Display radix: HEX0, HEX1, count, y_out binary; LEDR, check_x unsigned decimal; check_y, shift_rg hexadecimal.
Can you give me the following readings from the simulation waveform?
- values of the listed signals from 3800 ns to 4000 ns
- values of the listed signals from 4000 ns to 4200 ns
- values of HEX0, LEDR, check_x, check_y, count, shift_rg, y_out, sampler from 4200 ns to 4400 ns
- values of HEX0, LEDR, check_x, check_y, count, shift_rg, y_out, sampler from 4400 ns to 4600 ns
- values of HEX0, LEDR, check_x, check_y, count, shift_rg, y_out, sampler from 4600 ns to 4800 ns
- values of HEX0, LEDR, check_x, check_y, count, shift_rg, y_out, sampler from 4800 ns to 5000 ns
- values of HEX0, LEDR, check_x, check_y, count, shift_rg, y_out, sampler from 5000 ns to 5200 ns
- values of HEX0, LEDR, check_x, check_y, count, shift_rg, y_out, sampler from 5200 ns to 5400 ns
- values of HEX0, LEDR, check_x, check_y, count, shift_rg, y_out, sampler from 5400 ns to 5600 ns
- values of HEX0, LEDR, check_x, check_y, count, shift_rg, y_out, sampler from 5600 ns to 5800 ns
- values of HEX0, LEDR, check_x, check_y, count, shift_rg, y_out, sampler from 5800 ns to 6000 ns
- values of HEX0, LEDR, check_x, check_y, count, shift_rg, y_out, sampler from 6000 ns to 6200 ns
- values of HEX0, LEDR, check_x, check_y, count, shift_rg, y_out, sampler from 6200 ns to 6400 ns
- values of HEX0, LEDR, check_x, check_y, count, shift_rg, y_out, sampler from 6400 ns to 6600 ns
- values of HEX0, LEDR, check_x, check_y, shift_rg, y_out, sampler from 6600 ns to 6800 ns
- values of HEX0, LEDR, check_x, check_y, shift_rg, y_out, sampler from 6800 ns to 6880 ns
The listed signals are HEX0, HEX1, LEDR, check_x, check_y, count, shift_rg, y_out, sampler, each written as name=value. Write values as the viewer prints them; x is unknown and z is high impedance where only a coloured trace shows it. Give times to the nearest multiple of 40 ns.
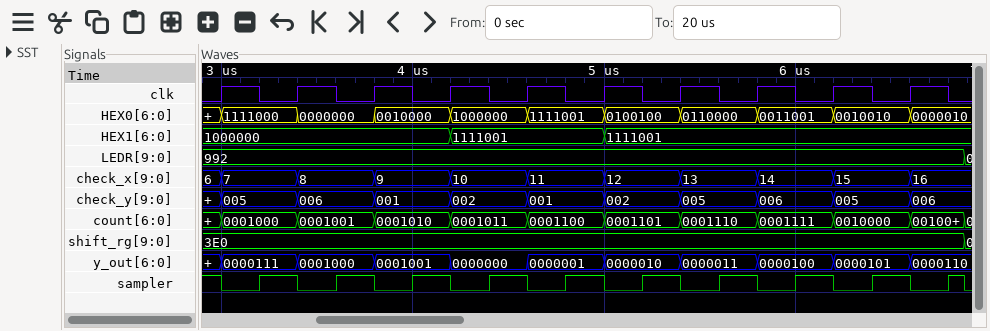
HEX0=0010000, HEX1=1000000, LEDR=992, check_x=9, check_y=001, count=0001010, shift_rg=3E0, y_out=0001001, sampler=0
HEX0=0010000, HEX1=1000000, LEDR=992, check_x=9, check_y=001, count=0001010, shift_rg=3E0, y_out=0001001, sampler=1
HEX0=1000000, LEDR=992, check_x=10, check_y=002, count=0001011, shift_rg=3E0, y_out=0000000, sampler=0
HEX0=1000000, LEDR=992, check_x=10, check_y=002, count=0001011, shift_rg=3E0, y_out=0000000, sampler=1
HEX0=1111001, LEDR=992, check_x=11, check_y=001, count=0001100, shift_rg=3E0, y_out=0000001, sampler=0
HEX0=1111001, LEDR=992, check_x=11, check_y=001, count=0001100, shift_rg=3E0, y_out=0000001, sampler=1
HEX0=0100100, LEDR=992, check_x=12, check_y=002, count=0001101, shift_rg=3E0, y_out=0000010, sampler=0
HEX0=0100100, LEDR=992, check_x=12, check_y=002, count=0001101, shift_rg=3E0, y_out=0000010, sampler=1
HEX0=0110000, LEDR=992, check_x=13, check_y=005, count=0001110, shift_rg=3E0, y_out=0000011, sampler=0
HEX0=0110000, LEDR=992, check_x=13, check_y=005, count=0001110, shift_rg=3E0, y_out=0000011, sampler=1
HEX0=0011001, LEDR=992, check_x=14, check_y=006, count=0001111, shift_rg=3E0, y_out=0000100, sampler=0
HEX0=0011001, LEDR=992, check_x=14, check_y=006, count=0001111, shift_rg=3E0, y_out=0000100, sampler=1
HEX0=0010010, LEDR=992, check_x=15, check_y=005, count=0010000, shift_rg=3E0, y_out=0000101, sampler=0
HEX0=0010010, LEDR=992, check_x=15, check_y=005, count=0010000, shift_rg=3E0, y_out=0000101, sampler=1
HEX0=0000010, LEDR=992, check_x=16, check_y=006, shift_rg=3E0, y_out=0000110, sampler=0
HEX0=0000010, LEDR=992, check_x=16, check_y=006, shift_rg=3E0, y_out=0000110, sampler=1
